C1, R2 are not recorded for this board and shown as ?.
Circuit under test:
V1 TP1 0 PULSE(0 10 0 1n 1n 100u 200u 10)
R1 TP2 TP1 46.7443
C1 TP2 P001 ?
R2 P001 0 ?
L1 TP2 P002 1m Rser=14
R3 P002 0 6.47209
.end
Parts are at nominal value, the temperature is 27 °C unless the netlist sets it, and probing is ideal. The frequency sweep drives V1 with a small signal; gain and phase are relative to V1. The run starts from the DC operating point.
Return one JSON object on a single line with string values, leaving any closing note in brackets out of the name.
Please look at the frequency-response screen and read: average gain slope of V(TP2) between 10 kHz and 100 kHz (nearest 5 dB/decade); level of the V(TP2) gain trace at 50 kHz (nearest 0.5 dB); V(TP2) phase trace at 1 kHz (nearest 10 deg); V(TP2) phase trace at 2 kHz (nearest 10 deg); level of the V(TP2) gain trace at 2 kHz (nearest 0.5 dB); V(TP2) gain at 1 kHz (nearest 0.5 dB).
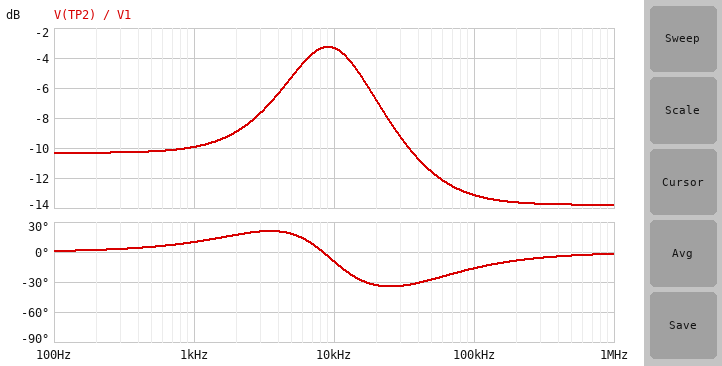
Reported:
{"average gain slope of V(TP2) between 10 kHz and 100 kHz": "-10 dB/decade", "level of the V(TP2) gain trace at 50 kHz": "-11.5 dB", "V(TP2) phase trace at 1 kHz": "10 deg", "V(TP2) phase trace at 2 kHz": "20 deg", "level of the V(TP2) gain trace at 2 kHz": "-9.0 dB", "V(TP2) gain at 1 kHz": "-10.0 dB"}
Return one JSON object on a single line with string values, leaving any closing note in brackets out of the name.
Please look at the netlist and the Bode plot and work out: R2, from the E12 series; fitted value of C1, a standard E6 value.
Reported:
{"R2, from the E12 series": "12 Ω", "fitted value of C1, a standard E6 value": "330 nF"}
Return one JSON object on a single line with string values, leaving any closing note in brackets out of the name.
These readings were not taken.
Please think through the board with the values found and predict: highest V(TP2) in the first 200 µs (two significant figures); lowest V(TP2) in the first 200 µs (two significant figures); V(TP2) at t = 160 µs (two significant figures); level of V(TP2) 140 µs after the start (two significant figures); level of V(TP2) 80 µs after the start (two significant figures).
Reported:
{"highest V(TP2) in the first 200 µs": "5.5 V", "lowest V(TP2) in the first 200 µs": "-2.5 V", "V(TP2) at t = 160 µs": "-470 mV", "level of V(TP2) 140 µs after the start": "-1.6 V", "level of V(TP2) 80 µs after the start": "3.0 V"}
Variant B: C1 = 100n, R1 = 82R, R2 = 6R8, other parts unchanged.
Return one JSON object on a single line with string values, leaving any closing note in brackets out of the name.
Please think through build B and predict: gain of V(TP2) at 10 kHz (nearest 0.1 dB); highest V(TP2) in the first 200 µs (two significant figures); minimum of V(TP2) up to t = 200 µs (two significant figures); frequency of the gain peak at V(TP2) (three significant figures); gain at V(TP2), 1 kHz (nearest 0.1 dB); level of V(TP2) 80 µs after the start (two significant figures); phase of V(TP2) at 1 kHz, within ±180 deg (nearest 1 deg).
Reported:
{"gain of V(TP2) at 10 kHz": "-3.8 dB", "highest V(TP2) in the first 200 µs": "5.9 V", "minimum of V(TP2) up to t = 200 µs": "-3.9 V", "frequency of the gain peak at V(TP2)": "16.9 kHz", "gain at V(TP2), 1 kHz": "-13.6 dB", "level of V(TP2) 80 µs after the start": "2.0 V", "phase of V(TP2) at 1 kHz, within ±180 deg": "13 deg"}
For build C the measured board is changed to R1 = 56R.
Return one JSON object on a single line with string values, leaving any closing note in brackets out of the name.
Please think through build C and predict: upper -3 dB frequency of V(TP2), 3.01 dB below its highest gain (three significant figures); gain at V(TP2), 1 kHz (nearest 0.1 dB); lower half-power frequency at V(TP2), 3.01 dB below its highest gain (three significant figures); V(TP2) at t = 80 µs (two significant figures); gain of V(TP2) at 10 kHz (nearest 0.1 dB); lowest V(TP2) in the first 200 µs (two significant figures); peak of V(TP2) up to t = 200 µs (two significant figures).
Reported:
{"upper -3 dB frequency of V(TP2), 3.01 dB below its highest gain": "17.3 kHz", "gain at V(TP2), 1 kHz": "-11.0 dB", "lower half-power frequency at V(TP2), 3.01 dB below its highest gain": "4.38 kHz", "V(TP2) at t = 80 µs": "2.6 V", "gain of V(TP2) at 10 kHz": "-3.9 dB", "lowest V(TP2) in the first 200 µs": "-2.4 V", "peak of V(TP2) up to t = 200 µs": "5.0 V"}
